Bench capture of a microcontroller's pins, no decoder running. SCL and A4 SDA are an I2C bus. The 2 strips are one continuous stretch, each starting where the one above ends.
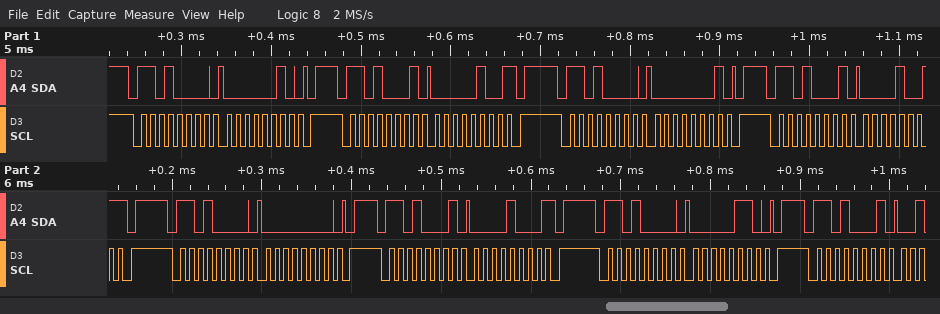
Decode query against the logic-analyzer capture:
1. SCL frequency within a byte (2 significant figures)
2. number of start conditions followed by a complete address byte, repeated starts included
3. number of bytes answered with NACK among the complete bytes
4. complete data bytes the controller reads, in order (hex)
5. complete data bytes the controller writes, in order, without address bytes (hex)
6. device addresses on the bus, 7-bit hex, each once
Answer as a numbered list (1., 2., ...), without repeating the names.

1. 100 kHz
2. 8
3. 3
4. 04 09 08
5. 02 01 00 06
6. 0x68
